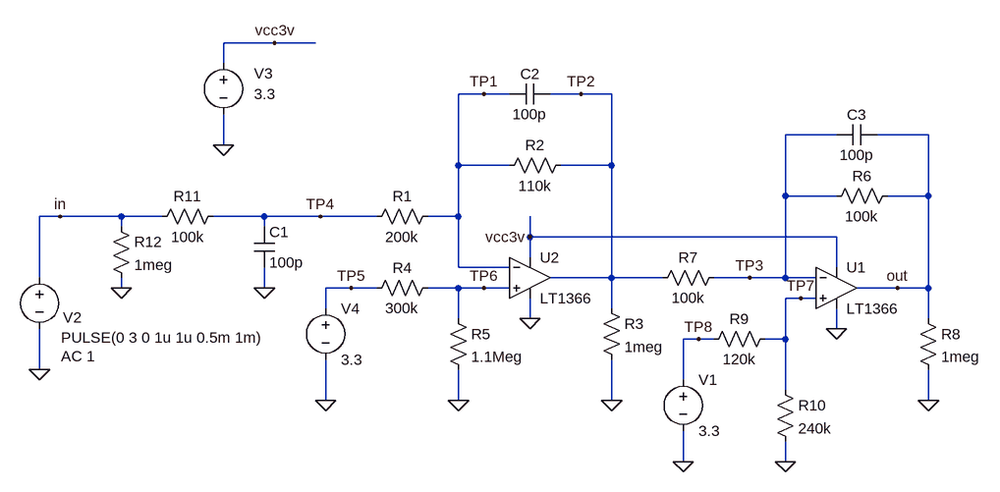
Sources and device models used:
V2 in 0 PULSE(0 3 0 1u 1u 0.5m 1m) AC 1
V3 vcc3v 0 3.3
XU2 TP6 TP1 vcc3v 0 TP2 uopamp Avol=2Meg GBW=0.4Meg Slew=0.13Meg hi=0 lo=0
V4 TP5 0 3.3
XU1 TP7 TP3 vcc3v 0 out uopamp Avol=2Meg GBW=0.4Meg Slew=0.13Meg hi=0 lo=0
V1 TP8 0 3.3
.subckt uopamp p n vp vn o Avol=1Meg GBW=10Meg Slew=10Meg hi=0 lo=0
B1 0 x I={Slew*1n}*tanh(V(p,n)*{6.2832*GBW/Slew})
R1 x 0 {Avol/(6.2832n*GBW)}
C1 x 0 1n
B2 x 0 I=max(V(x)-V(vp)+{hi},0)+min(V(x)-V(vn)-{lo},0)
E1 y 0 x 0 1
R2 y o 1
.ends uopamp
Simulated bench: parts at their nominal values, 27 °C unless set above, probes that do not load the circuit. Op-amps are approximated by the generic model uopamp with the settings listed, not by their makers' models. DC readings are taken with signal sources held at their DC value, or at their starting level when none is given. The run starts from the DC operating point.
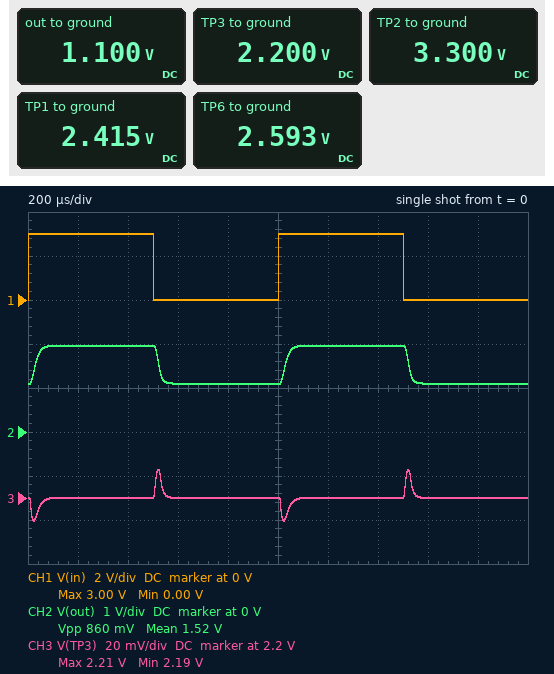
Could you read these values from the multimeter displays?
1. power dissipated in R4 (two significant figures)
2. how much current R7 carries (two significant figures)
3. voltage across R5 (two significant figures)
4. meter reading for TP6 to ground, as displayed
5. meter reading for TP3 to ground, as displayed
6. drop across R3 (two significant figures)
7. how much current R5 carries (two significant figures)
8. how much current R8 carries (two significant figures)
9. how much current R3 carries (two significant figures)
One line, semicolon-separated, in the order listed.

1.7 µW; 11 µA; 2.6 V; 2.593 V; 2.200 V; 3.3 V; 2.4 µA; 1.1 µA; 3.3 µA
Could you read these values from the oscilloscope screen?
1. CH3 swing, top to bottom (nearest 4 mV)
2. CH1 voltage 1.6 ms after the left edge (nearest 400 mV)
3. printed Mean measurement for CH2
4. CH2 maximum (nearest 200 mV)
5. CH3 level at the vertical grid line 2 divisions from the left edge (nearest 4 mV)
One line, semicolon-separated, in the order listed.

24 mV; 0 V; 1.52 V; 2.0 V; 2.200 V
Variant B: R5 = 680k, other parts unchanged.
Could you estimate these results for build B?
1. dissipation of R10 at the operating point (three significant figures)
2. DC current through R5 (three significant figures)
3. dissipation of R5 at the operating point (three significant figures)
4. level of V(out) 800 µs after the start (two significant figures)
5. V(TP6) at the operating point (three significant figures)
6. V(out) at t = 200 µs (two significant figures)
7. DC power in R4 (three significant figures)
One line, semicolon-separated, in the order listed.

20.2 µW; 3.37 µA; 7.71 µW; 1.3 V; 2.29 V; 2.4 V; 3.40 µW
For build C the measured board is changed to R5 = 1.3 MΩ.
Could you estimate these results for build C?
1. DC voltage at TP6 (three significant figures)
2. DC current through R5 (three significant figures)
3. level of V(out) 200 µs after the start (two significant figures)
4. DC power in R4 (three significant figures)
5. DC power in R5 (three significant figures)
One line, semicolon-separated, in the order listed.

2.68 V; 2.06 µA; 1.8 V; 1.28 µW; 5.53 µW
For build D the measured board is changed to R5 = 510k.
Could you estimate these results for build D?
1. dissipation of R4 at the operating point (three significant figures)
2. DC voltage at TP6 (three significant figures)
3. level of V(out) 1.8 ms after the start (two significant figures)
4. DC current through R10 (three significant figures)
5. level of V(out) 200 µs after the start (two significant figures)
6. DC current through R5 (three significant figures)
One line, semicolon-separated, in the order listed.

4.98 µW; 2.08 V; 1.6 V; 9.17 µA; 2.7 V; 4.07 µA
